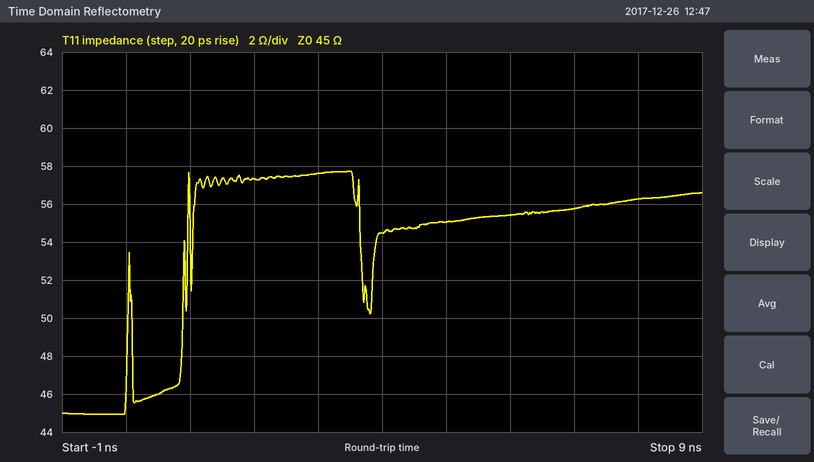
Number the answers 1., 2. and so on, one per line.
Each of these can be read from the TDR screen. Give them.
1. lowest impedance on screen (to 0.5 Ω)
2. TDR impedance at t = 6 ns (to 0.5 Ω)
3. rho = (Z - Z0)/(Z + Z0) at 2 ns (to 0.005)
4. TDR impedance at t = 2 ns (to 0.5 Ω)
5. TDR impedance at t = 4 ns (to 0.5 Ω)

1. 45.0 Ω
2. 55.5 Ω
3. +0.120
4. 57.5 Ω
5. 54.5 Ω
